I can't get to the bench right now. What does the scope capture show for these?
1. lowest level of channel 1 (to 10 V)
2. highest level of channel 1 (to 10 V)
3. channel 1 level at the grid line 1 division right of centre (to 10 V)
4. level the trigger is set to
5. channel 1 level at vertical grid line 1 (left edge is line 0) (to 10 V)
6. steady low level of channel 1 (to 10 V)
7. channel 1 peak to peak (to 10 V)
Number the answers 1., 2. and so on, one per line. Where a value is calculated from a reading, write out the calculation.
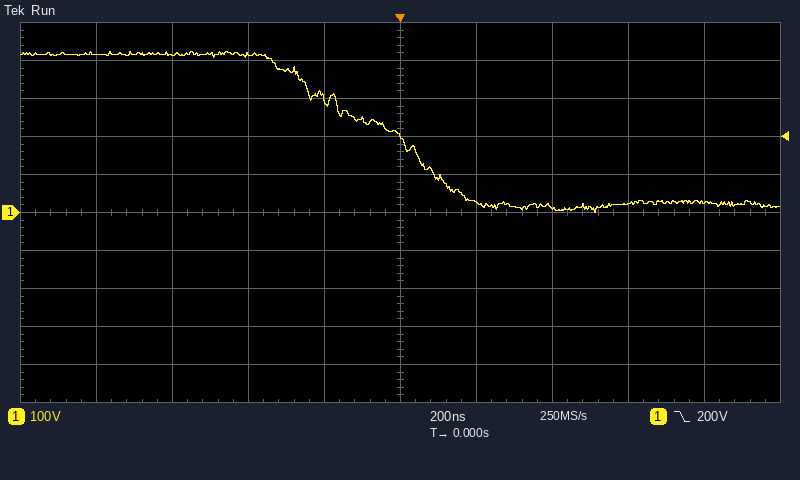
1. 0 V
2. 420 V
3. 30 V
4. 200 V
5. 420 V
6. 20 V
7. 420 V − (0 V) = 420 V
